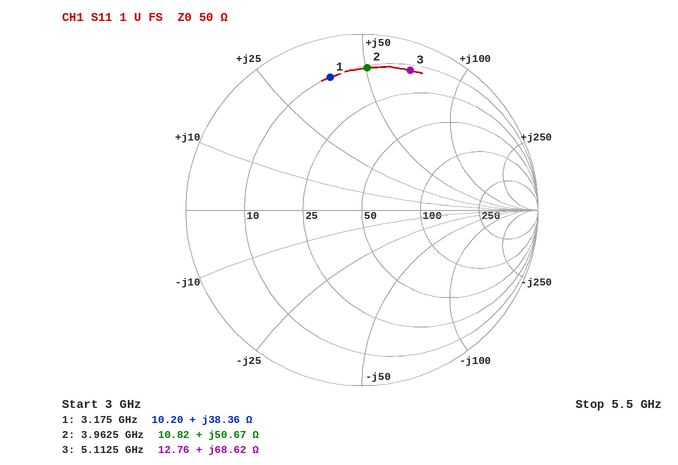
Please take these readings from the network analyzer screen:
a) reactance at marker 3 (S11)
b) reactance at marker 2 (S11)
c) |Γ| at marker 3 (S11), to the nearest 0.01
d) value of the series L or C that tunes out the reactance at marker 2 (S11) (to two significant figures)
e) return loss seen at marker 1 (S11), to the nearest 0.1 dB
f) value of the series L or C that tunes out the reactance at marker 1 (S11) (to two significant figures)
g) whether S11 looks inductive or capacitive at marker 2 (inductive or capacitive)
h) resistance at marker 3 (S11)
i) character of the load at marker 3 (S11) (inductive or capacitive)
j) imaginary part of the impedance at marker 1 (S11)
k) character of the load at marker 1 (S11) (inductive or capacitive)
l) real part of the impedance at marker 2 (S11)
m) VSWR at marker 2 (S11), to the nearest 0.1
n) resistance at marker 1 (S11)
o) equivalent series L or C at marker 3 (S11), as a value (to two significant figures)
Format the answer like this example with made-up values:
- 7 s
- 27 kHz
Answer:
- +68.62 Ω
- +50.67 Ω
- 0.84
- 790 fF
- 2.2 dB
- 1.3 pF
- inductive
- 12.76 Ω
- inductive
- +38.36 Ω
- inductive
- 10.82 Ω
- 9.5
- 10.20 Ω
- 2.1 nH
